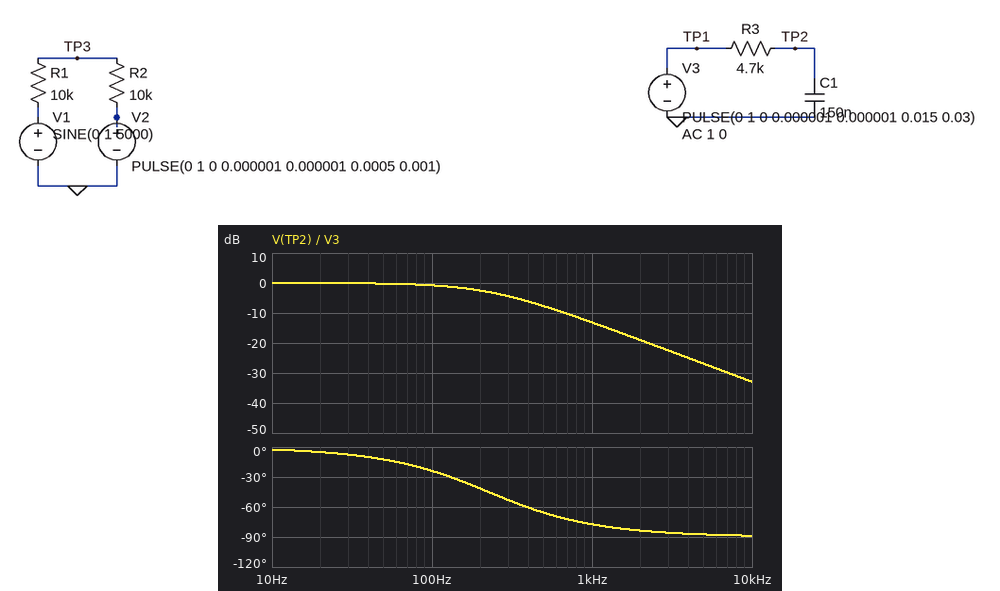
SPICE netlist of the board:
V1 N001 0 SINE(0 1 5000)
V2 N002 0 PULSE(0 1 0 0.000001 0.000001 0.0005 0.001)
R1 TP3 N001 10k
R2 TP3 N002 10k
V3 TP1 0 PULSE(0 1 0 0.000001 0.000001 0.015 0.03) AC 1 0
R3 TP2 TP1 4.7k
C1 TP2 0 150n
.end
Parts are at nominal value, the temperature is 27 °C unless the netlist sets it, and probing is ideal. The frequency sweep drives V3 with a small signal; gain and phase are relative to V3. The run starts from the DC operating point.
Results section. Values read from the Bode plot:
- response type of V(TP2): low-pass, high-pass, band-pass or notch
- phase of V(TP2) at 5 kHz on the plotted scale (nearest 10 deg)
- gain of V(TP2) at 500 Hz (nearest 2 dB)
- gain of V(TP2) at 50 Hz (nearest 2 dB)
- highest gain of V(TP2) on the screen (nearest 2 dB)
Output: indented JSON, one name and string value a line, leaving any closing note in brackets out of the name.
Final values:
{
  "response type of V(TP2): low-pass, high-pass, band-pass or notch": "low-pass",
  "phase of V(TP2) at 5 kHz on the plotted scale": "-90 deg",
  "gain of V(TP2) at 500 Hz": "-8 dB",
  "gain of V(TP2) at 50 Hz": "0 dB",
  "highest gain of V(TP2) on the screen": "0 dB"
}
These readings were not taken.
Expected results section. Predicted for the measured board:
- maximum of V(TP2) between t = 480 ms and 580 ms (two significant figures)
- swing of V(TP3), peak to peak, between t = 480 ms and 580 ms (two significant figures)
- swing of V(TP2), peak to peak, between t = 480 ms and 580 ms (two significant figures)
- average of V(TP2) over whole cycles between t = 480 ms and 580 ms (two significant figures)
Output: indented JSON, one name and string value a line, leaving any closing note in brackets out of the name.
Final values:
{
  "maximum of V(TP2) between t = 480 ms and 580 ms": "1.0 V",
  "swing of V(TP3), peak to peak, between t = 480 ms and 580 ms": "1.5 V",
  "swing of V(TP2), peak to peak, between t = 480 ms and 580 ms": "1.0 V",
  "average of V(TP2) over whole cycles between t = 480 ms and 580 ms": "500 mV"
}
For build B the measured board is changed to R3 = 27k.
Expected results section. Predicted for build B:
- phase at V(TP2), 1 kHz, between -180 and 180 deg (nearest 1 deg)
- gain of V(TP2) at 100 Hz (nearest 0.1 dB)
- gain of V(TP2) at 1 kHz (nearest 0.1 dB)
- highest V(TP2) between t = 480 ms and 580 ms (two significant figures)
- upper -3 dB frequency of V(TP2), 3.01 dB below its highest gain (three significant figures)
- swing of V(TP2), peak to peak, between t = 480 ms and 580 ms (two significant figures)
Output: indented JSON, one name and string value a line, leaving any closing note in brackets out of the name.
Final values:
{
  "phase at V(TP2), 1 kHz, between -180 and 180 deg": "-88 deg",
  "gain of V(TP2) at 100 Hz": "-8.7 dB",
  "gain of V(TP2) at 1 kHz": "-28.1 dB",
  "highest V(TP2) between t = 480 ms and 580 ms": "980 mV",
  "upper -3 dB frequency of V(TP2), 3.01 dB below its highest gain": "39.3 Hz",
  "swing of V(TP2), peak to peak, between t = 480 ms and 580 ms": "950 mV"
}
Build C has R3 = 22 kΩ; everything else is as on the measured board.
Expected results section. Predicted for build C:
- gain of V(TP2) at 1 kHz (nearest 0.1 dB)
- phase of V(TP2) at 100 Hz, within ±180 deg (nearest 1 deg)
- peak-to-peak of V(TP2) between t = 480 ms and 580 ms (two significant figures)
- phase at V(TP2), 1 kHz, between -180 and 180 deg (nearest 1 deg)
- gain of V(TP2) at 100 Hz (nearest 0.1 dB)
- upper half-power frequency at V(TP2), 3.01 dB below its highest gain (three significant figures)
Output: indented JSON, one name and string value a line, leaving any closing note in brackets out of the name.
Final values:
{
  "gain of V(TP2) at 1 kHz": "-26.3 dB",
  "phase of V(TP2) at 100 Hz, within ±180 deg": "-64 deg",
  "peak-to-peak of V(TP2) between t = 480 ms and 580 ms": "980 mV",
  "phase at V(TP2), 1 kHz, between -180 and 180 deg": "-87 deg",
  "gain of V(TP2) at 100 Hz": "-7.2 dB",
  "upper half-power frequency at V(TP2), 3.01 dB below its highest gain": "48.2 Hz"
}
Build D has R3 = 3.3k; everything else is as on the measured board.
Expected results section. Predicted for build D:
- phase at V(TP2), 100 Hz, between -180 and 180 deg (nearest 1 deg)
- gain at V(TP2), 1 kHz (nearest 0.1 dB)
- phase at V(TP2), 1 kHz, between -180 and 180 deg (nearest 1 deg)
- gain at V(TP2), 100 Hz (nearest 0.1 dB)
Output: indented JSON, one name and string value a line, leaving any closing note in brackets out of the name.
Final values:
{
  "phase at V(TP2), 100 Hz, between -180 and 180 deg": "-17 deg",
  "gain at V(TP2), 1 kHz": "-10.3 dB",
  "phase at V(TP2), 1 kHz, between -180 and 180 deg": "-72 deg",
  "gain at V(TP2), 100 Hz": "-0.4 dB"
}
